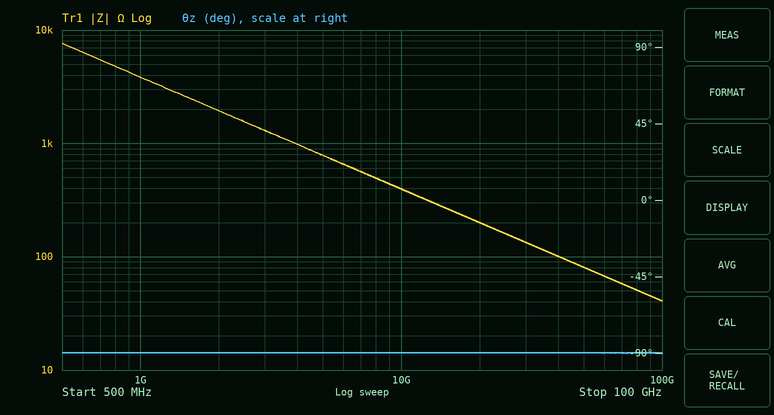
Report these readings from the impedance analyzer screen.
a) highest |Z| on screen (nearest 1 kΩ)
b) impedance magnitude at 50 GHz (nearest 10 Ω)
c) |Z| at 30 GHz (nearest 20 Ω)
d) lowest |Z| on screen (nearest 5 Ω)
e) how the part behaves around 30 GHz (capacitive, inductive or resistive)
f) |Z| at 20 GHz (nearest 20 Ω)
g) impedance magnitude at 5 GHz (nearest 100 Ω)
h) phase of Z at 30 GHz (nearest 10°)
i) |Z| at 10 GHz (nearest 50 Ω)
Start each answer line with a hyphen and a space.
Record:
- 8 kΩ
- 80 Ω
- 140 Ω
- 40 Ω
- capacitive
- 200 Ω
- 800 Ω
- -90°
- 400 Ω
